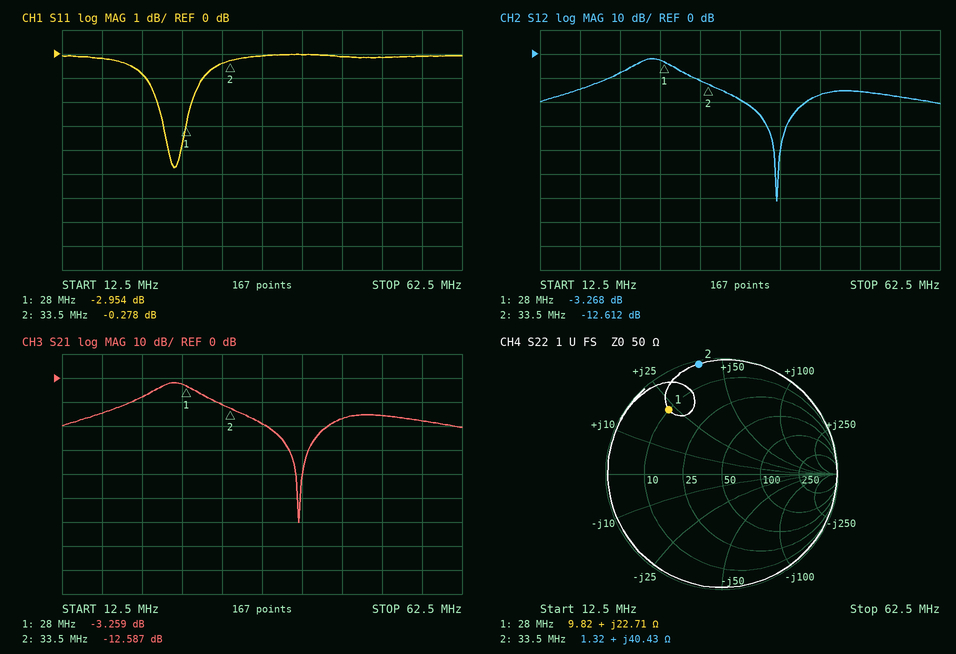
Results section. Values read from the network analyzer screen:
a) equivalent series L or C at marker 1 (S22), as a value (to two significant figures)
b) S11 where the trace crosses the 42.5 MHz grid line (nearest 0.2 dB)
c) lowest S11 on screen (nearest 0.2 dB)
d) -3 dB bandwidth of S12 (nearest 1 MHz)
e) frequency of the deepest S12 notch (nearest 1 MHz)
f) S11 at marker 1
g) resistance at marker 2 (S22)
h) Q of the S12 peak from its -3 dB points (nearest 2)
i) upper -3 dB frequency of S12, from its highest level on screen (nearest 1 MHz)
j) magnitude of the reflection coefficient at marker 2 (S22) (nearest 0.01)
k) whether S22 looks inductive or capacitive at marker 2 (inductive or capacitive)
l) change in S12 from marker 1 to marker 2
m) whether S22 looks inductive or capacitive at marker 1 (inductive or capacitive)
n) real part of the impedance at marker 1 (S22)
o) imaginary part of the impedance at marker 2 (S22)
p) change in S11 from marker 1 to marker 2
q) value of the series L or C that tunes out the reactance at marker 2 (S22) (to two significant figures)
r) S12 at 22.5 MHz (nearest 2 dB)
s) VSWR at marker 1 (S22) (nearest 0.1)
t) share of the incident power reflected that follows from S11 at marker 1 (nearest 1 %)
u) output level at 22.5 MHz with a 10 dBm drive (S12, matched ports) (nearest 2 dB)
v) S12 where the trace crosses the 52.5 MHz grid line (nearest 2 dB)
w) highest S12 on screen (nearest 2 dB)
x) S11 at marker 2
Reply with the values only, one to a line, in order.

130 nH
0.0 dB
-4.8 dB
5 MHz
42 MHz
-2.954 dB
1.32 Ω
6
29 MHz
0.97
inductive
-9.344 dB
inductive
9.82 Ω
+40.43 Ω
2.676 dB
120 pF
-8 dB
6.2
51 %
2 dBm
-16 dB
-2 dB
-0.278 dB
